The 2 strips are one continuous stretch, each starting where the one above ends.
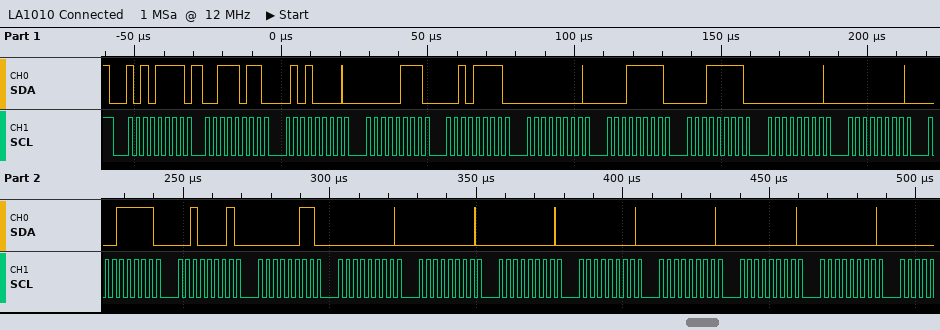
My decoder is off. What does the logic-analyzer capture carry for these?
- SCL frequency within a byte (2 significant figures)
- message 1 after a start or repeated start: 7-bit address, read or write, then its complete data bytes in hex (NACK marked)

400 kHz
0x57 read: 3B 50 07 2F 00 1F 1F 00 00 1F 21 03 00 00 00 00 00 00 00
